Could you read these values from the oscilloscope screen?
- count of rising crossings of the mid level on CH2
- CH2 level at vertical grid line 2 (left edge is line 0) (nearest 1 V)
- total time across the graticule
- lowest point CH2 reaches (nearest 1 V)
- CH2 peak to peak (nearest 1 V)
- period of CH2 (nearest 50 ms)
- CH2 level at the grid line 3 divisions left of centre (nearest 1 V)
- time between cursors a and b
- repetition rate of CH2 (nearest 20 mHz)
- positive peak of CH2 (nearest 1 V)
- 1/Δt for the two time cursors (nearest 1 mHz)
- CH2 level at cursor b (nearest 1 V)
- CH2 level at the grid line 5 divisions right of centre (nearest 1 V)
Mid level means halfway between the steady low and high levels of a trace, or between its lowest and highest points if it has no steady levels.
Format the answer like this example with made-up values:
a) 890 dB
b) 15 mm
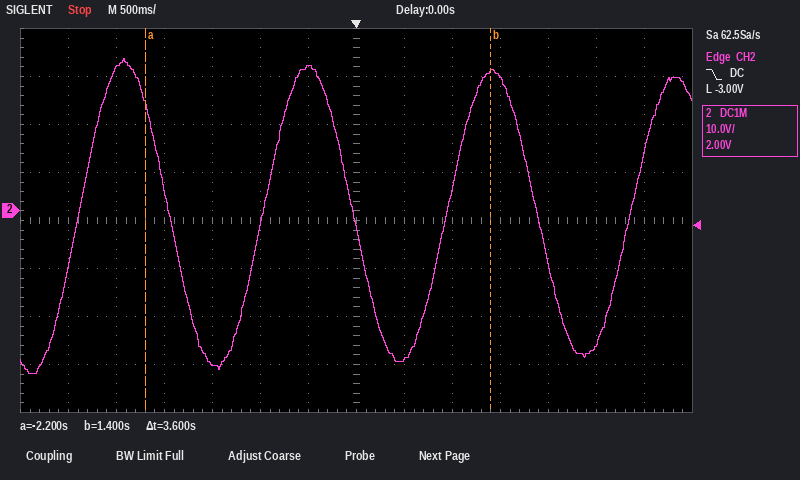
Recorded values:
a) 4
b) 30 V
c) 7 s
d) -34 V
e) 66 V
f) 1.90 s
g) -32 V
h) 3.6 s
i) 520 mHz
j) 32 V
k) 278 mHz
l) 29 V
m) -28 V
